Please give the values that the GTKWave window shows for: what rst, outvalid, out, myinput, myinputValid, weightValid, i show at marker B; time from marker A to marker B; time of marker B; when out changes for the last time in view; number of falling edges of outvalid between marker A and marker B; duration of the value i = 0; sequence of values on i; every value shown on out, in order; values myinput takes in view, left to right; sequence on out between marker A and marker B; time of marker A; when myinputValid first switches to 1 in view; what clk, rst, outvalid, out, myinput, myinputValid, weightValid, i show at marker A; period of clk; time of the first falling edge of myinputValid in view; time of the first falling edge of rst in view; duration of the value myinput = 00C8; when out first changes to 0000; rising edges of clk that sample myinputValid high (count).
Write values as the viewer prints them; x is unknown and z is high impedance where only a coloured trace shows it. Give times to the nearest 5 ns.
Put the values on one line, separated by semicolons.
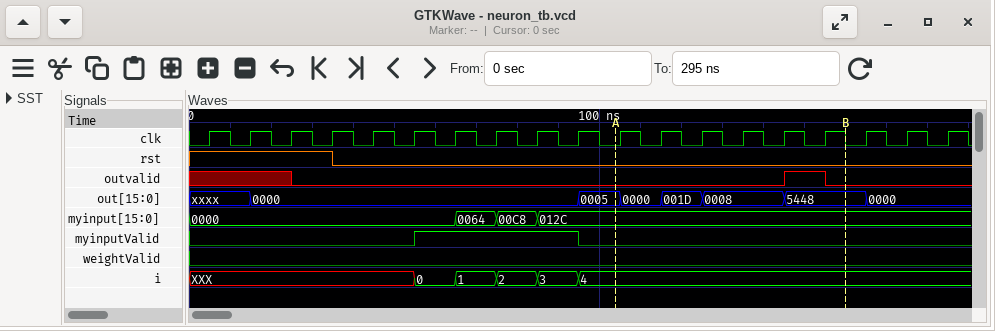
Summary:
rst=0, outvalid=0, out=5448, myinput=012C, myinputValid=0, weightValid=0, i=4; 55 ns; 160 ns; 165 ns; 1; 10 ns; XXX, 0, 1, 2, 3, 4; xxxx, 0000, 0005, 0000, 001D, 0008, 5448, 0000; 0000, 0064, 00C8, 012C; 0005, 0000, 001D, 0008, 5448; 105 ns; 55 ns; clk=0, rst=0, outvalid=0, out=0005, myinput=012C, myinputValid=0, weightValid=0, i=4; 10 ns; 95 ns; 35 ns; 10 ns; 15 ns; 4
